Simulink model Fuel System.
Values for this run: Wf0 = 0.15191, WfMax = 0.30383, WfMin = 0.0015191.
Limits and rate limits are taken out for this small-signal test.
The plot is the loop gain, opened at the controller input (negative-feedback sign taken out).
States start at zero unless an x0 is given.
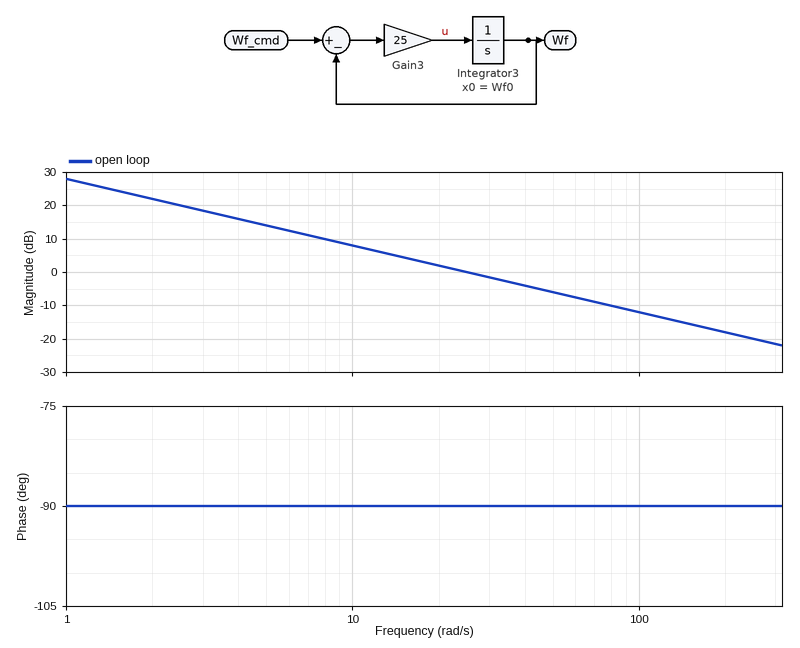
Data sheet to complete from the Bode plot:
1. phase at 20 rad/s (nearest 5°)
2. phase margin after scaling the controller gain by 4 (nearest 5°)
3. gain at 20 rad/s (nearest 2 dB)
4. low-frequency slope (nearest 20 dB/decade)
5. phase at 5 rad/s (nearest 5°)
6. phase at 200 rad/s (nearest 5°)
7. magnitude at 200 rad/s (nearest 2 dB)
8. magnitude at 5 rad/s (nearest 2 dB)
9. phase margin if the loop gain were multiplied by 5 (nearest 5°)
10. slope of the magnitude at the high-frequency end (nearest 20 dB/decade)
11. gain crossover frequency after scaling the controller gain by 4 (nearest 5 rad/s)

-90°
90°
2 dB
-20 dB/decade
-90°
-90°
-18 dB
14 dB
90°
-20 dB/decade
100 rad/s
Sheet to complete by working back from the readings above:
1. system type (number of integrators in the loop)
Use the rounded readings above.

1
